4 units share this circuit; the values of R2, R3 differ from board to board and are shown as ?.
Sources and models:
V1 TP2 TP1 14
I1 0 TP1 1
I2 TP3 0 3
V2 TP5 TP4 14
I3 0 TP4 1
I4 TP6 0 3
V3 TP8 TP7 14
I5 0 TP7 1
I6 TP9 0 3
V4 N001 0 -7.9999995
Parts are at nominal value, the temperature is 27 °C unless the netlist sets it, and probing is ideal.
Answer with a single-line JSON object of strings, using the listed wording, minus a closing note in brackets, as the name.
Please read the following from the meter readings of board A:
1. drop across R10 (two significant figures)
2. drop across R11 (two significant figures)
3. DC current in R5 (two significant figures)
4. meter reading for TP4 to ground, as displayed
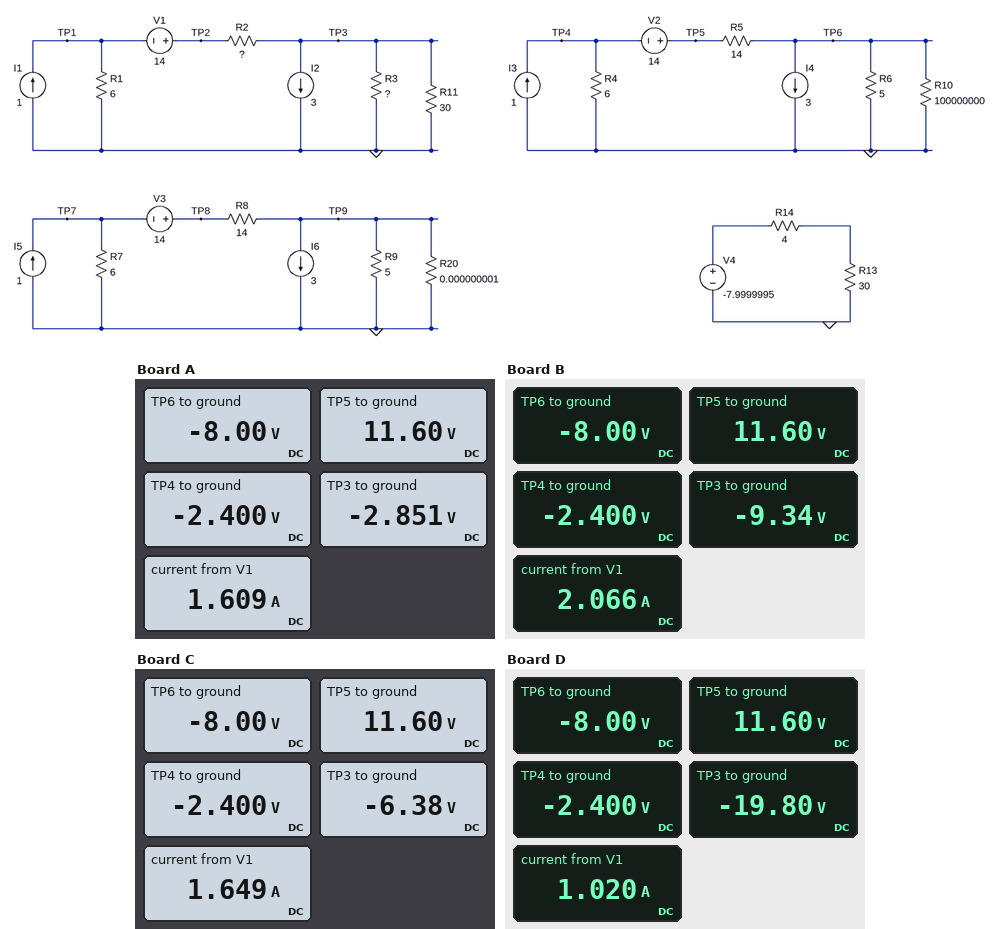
{"drop across R10": "8.0 V", "drop across R11": "2.9 V", "DC current in R5": "1.4 A", "meter reading for TP4 to ground, as displayed": "-2.400 V"}
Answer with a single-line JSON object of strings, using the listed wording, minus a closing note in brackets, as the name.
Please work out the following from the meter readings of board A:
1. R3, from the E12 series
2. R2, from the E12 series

{"R3, from the E12 series": "2.2 Ω", "R2, from the E12 series": "8.2 Ω"}
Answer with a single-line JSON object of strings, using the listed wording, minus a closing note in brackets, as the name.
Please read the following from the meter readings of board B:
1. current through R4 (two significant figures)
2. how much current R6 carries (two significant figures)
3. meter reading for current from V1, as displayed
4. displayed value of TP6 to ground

{"current through R4": "400 mA", "how much current R6 carries": "1.6 A", "meter reading for current from V1, as displayed": "2.066 A", "displayed value of TP6 to ground": "-8.00 V"}
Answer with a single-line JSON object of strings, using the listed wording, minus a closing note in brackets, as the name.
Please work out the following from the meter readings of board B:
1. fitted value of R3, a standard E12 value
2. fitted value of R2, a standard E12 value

{"fitted value of R3, a standard E12 value": "15 Ω", "fitted value of R2, a standard E12 value": "8.2 Ω"}
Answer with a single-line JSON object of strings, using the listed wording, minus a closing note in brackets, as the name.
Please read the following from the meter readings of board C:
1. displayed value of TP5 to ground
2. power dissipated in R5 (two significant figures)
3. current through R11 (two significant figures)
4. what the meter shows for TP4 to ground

{"displayed value of TP5 to ground": "11.60 V", "power dissipated in R5": "27 W", "current through R11": "210 mA", "what the meter shows for TP4 to ground": "-2.400 V"}
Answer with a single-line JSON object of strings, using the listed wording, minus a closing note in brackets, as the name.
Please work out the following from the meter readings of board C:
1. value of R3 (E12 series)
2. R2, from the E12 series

{"value of R3": "5.6 Ω", "R2, from the E12 series": "10 Ω"}
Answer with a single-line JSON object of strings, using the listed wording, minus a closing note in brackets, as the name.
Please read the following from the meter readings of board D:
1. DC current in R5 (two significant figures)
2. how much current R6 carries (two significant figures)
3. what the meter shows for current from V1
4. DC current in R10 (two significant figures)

{"DC current in R5": "1.4 A", "how much current R6 carries": "1.6 A", "what the meter shows for current from V1": "1.020 A", "DC current in R10": "80 nA"}
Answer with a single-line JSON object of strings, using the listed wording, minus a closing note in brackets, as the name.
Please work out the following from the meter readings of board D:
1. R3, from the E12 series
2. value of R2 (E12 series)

{"R3, from the E12 series": "15 Ω", "value of R2": "33 Ω"}
